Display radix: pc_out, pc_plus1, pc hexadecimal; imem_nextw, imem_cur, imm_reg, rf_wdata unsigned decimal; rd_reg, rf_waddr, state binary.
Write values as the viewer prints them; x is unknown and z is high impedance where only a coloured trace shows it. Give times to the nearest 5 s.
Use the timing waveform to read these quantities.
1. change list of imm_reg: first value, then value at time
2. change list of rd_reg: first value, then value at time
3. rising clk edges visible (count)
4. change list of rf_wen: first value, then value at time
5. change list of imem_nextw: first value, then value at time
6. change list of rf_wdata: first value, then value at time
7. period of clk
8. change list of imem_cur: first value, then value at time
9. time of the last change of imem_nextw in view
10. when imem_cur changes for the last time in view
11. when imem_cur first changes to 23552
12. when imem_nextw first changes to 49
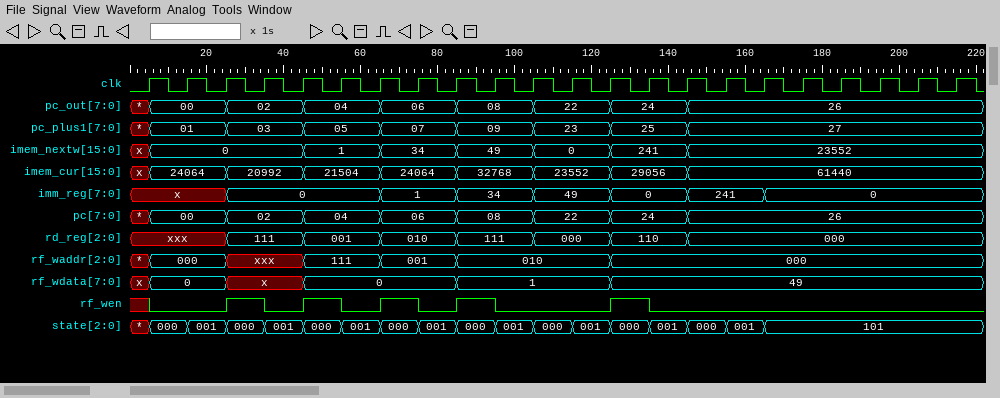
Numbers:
x, 0 at 25 s, 1 at 65 s, 34 at 85 s, 49 at 105 s, 0 at 125 s, 241 at 145 s, 0 at 165 s
xxx, 111 at 25 s, 001 at 45 s, 010 at 65 s, 111 at 85 s, 000 at 105 s, 110 at 125 s, 000 at 145 s
22
x, 0 at 5 s, 1 at 25 s, 0 at 35 s, 1 at 45 s, 0 at 55 s, 1 at 65 s, 0 at 75 s, 1 at 85 s, 0 at 95 s, 1 at 125 s, 0 at 135 s
x, 0 at 5 s, 1 at 45 s, 34 at 65 s, 49 at 85 s, 0 at 105 s, 241 at 125 s, 23552 at 145 s
x, 0 at 5 s, x at 25 s, 0 at 45 s, 1 at 85 s, 49 at 125 s
10 s
x, 24064 at 5 s, 20992 at 25 s, 21504 at 45 s, 24064 at 65 s, 32768 at 85 s, 23552 at 105 s, 29056 at 125 s, 61440 at 145 s
145 s
145 s
105 s
85 s
